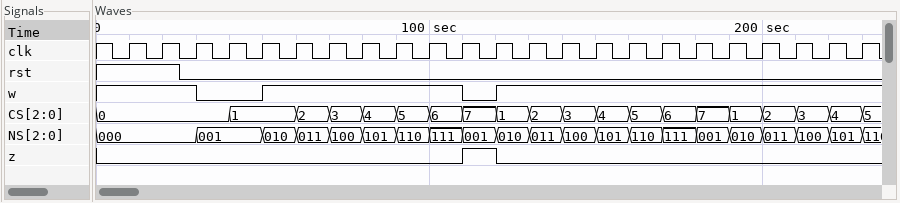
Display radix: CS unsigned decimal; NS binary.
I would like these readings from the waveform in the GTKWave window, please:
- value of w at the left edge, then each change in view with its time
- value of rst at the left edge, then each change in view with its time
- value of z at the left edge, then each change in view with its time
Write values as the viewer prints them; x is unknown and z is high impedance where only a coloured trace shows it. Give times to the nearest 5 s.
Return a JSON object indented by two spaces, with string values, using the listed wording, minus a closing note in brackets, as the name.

{
  "value of w at the left edge, then each change in view with its time": "1, 0 at 30 s, 1 at 50 s, 0 at 110 s, 1 at 120 s",
  "value of rst at the left edge, then each change in view with its time": "1, 0 at 25 s",
  "value of z at the left edge, then each change in view with its time": "0, 1 at 110 s, 0 at 120 s"
}
